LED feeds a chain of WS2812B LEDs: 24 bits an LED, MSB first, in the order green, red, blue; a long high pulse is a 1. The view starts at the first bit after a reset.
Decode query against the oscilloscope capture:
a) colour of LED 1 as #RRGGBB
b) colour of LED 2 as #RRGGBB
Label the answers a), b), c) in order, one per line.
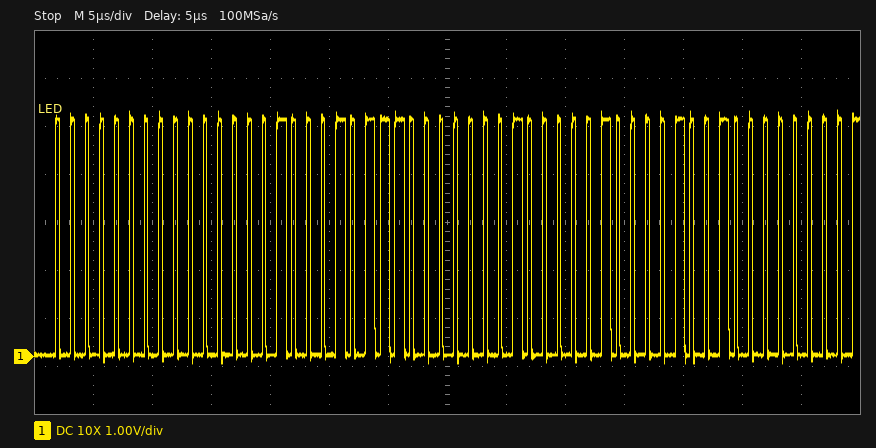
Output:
a) #010017
b) #040124
